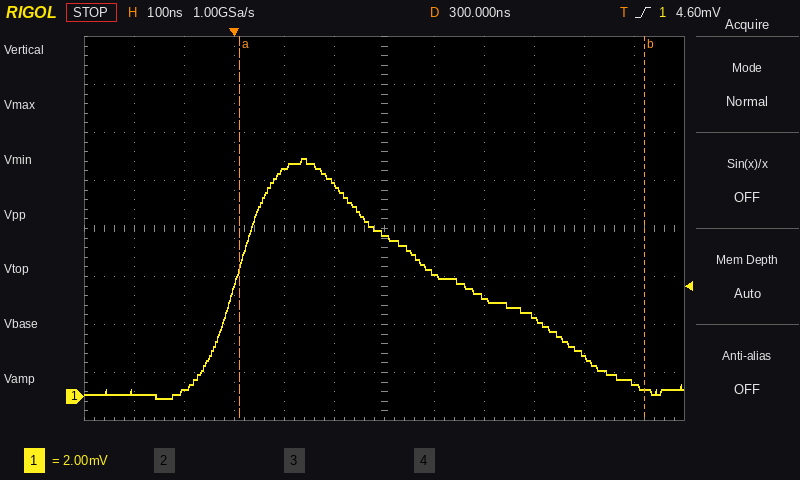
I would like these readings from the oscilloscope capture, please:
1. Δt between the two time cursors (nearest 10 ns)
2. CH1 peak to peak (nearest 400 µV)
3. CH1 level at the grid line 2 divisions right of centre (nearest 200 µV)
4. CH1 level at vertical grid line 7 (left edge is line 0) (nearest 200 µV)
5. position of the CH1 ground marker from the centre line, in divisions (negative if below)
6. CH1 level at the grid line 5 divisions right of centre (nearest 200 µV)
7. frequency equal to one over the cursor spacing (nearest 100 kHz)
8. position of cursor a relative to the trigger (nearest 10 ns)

810 ns
10.0 mV
4.2 mV
5.2 mV
-3.5 div
600 µV
1.2 MHz
+10 ns
